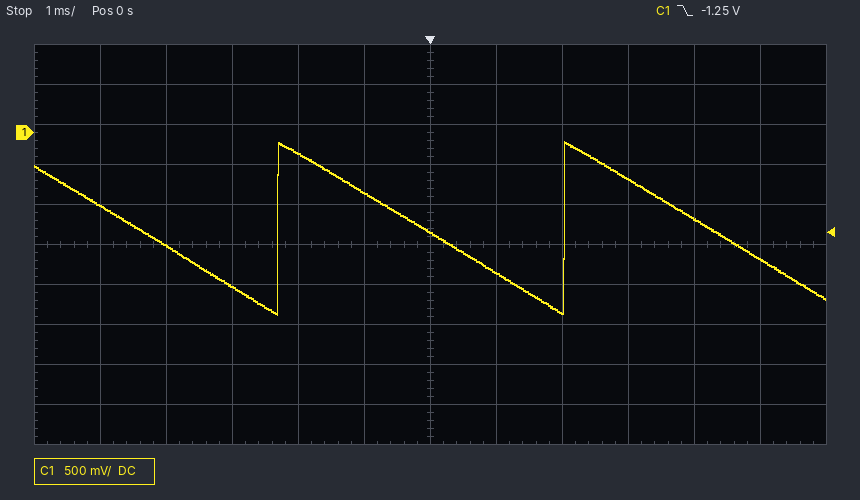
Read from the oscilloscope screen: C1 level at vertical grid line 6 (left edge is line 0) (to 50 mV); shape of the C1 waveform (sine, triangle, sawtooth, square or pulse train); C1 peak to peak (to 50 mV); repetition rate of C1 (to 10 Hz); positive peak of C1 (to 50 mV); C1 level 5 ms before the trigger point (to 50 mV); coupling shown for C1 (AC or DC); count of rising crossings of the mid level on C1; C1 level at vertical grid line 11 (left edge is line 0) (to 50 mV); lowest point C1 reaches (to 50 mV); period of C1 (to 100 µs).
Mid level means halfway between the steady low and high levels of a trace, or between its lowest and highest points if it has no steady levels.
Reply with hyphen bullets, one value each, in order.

- -1.25 V
- sawtooth
- 2.15 V
- 230 Hz
- -100 mV
- -900 mV
- DC
- 2
- -1.60 V
- -2.25 V
- 4.3 ms
